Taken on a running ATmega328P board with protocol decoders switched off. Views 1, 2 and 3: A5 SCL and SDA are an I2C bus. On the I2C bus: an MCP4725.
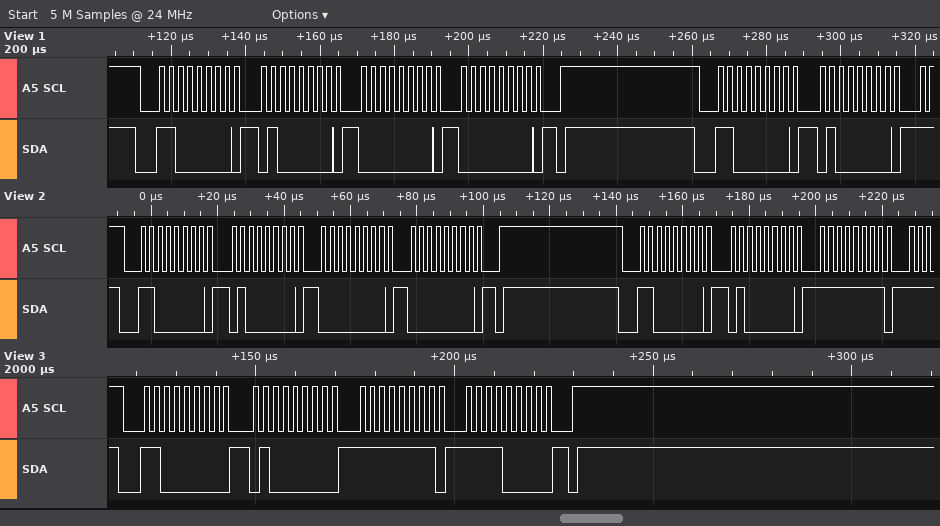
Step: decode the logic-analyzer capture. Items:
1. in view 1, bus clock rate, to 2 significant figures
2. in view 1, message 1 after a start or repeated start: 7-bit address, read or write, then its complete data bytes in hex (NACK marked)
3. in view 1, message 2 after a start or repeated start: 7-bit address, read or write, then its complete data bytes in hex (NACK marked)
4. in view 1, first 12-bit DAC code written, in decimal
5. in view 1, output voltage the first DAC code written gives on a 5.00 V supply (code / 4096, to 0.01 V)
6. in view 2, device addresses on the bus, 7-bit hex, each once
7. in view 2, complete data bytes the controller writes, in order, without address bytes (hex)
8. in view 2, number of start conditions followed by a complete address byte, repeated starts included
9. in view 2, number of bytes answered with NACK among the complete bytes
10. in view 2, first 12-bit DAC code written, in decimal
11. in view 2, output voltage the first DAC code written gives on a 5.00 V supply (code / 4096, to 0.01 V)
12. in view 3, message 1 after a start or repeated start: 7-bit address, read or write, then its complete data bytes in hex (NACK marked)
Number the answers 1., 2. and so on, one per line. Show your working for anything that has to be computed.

1. 400 kHz
2. 0x60 write: 40 00 00
3. 0x60 write: 40
4. 0
5. 0 / 4096 x 5.00 V = 0.00 V
6. 0x60
7. 40 00 00 40 FF
8. 2
9. 0
10. 0
11. 0 / 4096 x 5.00 V = 0.00 V
12. 0x60 write: 40 FF F0
